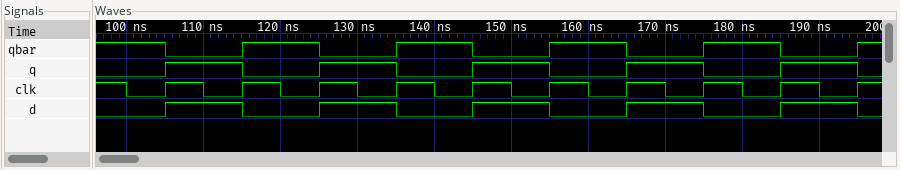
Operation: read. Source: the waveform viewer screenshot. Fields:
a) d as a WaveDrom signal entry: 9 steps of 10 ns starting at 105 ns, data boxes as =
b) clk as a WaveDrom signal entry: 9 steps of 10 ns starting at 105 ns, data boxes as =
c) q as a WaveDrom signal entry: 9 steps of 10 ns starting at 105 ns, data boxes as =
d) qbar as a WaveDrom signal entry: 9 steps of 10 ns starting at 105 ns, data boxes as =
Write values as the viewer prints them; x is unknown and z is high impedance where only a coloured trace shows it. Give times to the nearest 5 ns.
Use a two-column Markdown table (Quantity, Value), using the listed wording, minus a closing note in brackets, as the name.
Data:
| Quantity | Value |
|---|---|
| d as a WaveDrom signal entry: 9 steps of 10 ns starting at 105 ns, data boxes as = | {name: 'd', wave: '101010101'} |
| clk as a WaveDrom signal entry: 9 steps of 10 ns starting at 105 ns, data boxes as = | {name: 'clk', wave: 'p........'} |
| q as a WaveDrom signal entry: 9 steps of 10 ns starting at 105 ns, data boxes as = | {name: 'q', wave: '101010101'} |
| qbar as a WaveDrom signal entry: 9 steps of 10 ns starting at 105 ns, data boxes as = | {name: 'qbar', wave: '010101010'} |
